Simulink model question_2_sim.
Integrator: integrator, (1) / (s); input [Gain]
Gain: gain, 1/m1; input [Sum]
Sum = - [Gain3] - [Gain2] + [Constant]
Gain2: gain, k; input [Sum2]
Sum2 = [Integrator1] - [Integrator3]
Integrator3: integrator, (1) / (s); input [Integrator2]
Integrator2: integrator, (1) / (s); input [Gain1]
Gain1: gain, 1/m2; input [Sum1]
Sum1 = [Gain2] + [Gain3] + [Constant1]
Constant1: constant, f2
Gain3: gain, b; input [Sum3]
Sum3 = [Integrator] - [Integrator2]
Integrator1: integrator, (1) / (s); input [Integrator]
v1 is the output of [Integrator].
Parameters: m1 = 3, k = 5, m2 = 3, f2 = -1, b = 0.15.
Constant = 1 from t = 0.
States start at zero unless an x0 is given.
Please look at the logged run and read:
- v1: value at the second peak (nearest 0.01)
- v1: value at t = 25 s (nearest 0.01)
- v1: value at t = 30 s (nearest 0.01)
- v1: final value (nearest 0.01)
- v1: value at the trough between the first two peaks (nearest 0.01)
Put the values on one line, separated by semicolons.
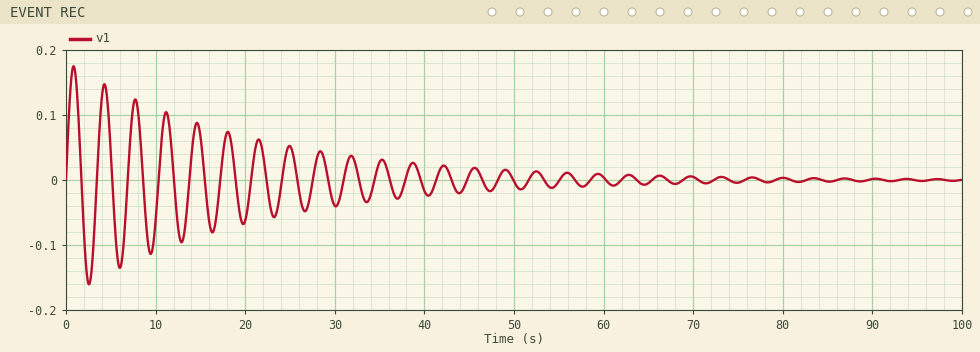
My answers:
0.15; 0.05; -0.04; 0.00; -0.16
